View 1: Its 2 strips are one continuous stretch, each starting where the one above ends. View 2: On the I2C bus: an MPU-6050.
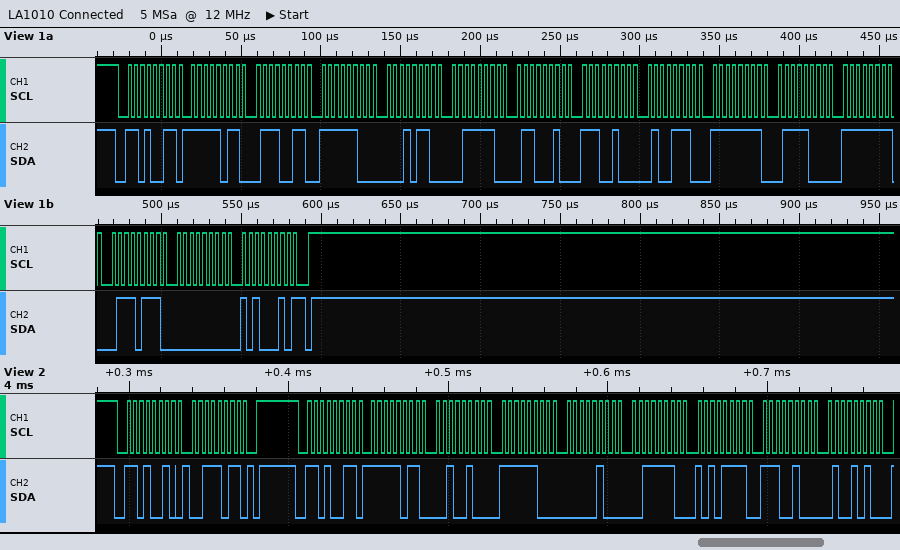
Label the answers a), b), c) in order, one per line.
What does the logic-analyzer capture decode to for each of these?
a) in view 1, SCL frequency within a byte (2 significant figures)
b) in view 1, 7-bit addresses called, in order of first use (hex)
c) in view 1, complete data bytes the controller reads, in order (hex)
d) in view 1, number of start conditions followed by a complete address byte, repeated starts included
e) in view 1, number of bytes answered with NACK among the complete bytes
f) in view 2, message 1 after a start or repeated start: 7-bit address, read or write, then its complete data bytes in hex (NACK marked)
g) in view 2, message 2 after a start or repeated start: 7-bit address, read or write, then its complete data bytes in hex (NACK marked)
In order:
a) 250 kHz
b) 0x69
c) FB 73 FC 16 3E 62 E4 4E FF 78 FF 77 00 A2
d) 1
e) 1
f) 0x69 write: 3B
g) 0x69 read: FB 24 FC 04 3E AF E4 4A
